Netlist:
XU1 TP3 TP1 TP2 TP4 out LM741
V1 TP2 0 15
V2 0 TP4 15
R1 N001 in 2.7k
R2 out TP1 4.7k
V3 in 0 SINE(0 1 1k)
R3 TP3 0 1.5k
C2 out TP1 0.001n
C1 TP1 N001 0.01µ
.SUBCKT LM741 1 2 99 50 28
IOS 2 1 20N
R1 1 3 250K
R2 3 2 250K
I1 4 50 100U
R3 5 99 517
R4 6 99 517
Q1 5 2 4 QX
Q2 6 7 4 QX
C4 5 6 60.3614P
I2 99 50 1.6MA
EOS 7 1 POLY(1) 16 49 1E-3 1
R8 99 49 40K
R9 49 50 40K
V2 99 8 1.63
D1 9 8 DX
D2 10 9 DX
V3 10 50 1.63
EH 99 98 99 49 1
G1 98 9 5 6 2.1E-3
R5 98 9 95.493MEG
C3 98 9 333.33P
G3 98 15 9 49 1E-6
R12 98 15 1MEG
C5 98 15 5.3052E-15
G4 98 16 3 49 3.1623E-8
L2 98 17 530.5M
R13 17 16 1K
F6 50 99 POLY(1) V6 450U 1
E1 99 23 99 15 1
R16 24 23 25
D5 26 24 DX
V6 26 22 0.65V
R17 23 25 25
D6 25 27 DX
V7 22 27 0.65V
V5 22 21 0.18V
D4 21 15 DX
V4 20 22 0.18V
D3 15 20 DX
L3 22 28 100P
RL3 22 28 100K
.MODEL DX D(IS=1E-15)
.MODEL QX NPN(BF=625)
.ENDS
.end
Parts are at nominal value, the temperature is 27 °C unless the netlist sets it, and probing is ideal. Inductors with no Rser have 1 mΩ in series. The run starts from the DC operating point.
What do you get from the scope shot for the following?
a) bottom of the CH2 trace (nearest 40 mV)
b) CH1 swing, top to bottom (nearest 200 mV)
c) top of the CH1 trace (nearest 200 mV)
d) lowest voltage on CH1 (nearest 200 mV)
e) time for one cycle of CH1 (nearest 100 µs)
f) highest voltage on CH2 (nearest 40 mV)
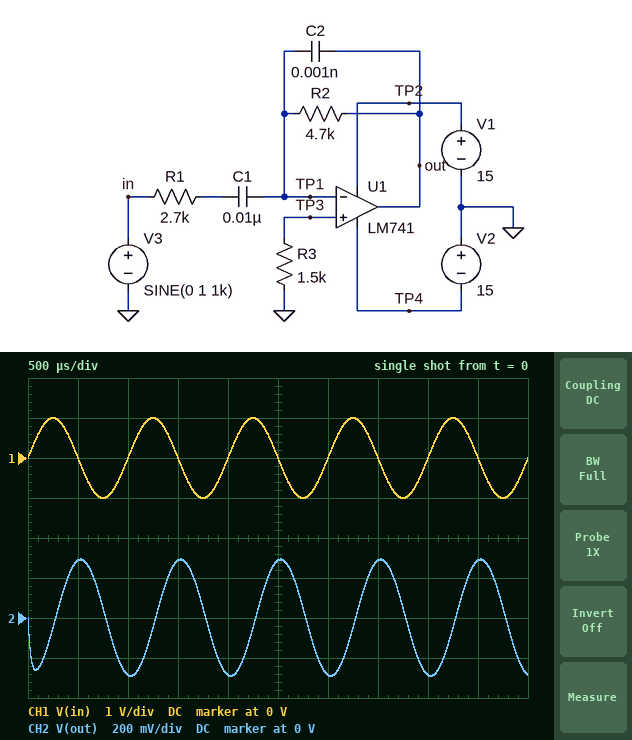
-280 mV
2.0 V
1.0 V
-1.0 V
1.0 ms
280 mV
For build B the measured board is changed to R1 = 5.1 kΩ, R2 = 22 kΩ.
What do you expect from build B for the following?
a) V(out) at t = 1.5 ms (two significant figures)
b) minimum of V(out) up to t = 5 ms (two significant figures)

1.3 V
-1.3 V
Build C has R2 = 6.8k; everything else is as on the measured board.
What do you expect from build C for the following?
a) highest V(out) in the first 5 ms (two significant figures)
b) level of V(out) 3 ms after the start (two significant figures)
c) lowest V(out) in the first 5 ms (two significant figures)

420 mV
-410 mV
-420 mV
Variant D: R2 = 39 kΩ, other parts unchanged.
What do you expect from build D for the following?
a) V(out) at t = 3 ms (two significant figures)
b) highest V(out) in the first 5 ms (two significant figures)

-2.4 V
2.4 V
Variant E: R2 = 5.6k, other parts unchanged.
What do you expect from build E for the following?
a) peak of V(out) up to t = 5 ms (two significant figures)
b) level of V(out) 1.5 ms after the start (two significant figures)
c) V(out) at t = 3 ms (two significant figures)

350 mV
340 mV
-340 mV
